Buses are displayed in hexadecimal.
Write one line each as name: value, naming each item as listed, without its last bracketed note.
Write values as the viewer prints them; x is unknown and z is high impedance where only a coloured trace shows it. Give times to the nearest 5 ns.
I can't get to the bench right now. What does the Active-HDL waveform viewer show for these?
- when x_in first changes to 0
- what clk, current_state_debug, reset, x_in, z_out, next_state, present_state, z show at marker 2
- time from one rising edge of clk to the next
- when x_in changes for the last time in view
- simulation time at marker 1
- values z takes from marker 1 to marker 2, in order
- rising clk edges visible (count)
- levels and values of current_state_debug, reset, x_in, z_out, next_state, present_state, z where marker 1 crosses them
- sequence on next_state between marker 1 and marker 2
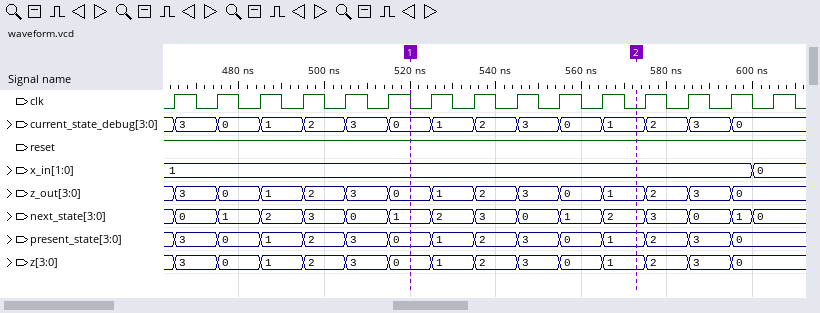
when x_in first changes to 0: 600 ns
what clk, current_state_debug, reset, x_in, z_out, next_state, present_state, z show at marker 2: clk=0, current_state_debug=1, reset=1, x_in=1, z_out=1, next_state=2, present_state=1, z=1
time from one rising edge of clk to the next: 10 ns
when x_in changes for the last time in view: 600 ns
simulation time at marker 1: 520 ns
values z takes from marker 1 to marker 2, in order: 0, 1, 2, 3, 0, 1
rising clk edges visible: 15
levels and values of current_state_debug, reset, x_in, z_out, next_state, present_state, z where marker 1 crosses them: current_state_debug=0, reset=1, x_in=1, z_out=0, next_state=1, present_state=0, z=0
sequence on next_state between marker 1 and marker 2: 1, 2, 3, 0, 1, 2
